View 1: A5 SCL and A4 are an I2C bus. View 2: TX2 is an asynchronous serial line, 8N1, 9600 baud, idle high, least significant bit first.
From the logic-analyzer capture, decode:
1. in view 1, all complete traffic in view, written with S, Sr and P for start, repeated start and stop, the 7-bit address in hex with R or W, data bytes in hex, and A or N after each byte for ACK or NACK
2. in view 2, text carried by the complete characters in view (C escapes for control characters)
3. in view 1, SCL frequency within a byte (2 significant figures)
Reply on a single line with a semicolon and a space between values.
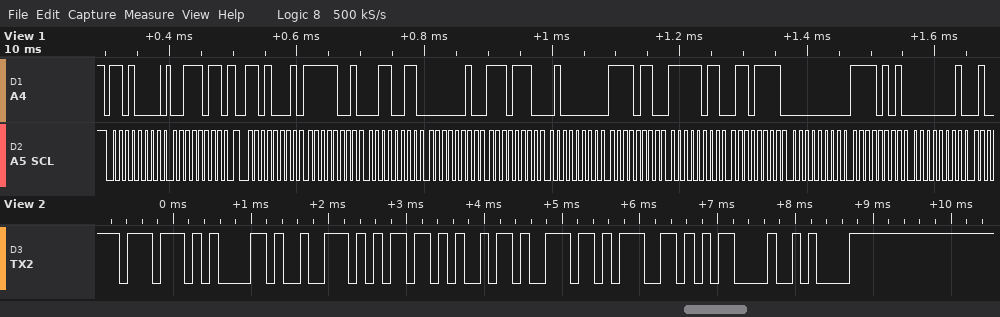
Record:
S 68W A 3B A Sr 68R A F9 A 33 A 02 A EE A 40 A F6 A FB A 6F A 00 A F5 A 01 A; "warming\r\n"; 100 kHz
